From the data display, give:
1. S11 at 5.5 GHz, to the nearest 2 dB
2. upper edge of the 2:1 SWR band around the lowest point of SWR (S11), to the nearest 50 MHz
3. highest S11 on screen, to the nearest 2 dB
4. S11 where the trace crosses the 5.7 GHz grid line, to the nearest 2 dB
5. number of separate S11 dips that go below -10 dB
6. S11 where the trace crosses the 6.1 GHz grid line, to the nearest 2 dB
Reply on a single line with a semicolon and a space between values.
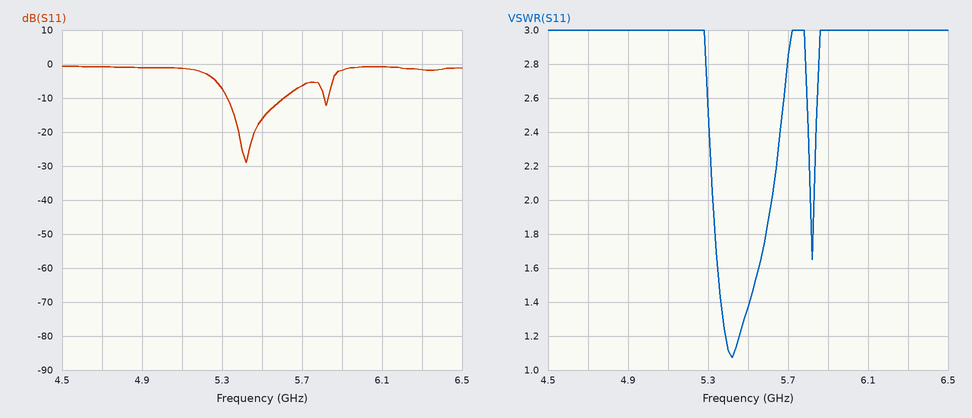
-16 dB; 5.60 GHz; 0 dB; -6 dB; 2; 0 dB
